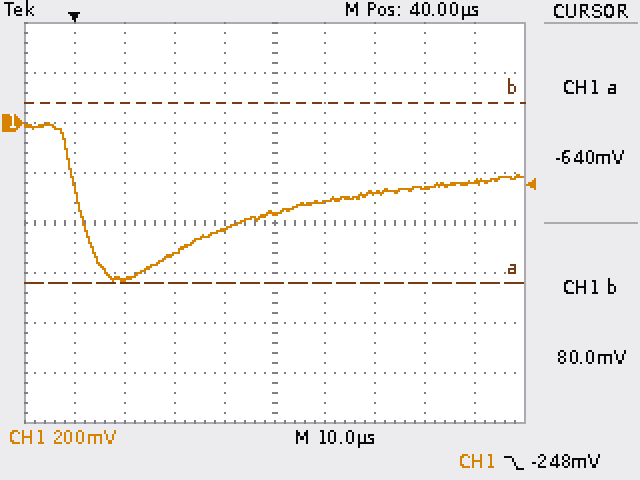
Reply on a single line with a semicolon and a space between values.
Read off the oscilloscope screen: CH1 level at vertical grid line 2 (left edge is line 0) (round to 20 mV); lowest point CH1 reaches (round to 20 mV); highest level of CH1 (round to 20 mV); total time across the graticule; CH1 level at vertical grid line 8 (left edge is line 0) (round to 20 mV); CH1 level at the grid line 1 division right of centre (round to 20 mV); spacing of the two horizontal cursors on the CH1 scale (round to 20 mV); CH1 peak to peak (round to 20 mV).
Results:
-620 mV; -640 mV; 0 mV; 100 µs; -260 mV; -320 mV; 720 mV; 640 mV
